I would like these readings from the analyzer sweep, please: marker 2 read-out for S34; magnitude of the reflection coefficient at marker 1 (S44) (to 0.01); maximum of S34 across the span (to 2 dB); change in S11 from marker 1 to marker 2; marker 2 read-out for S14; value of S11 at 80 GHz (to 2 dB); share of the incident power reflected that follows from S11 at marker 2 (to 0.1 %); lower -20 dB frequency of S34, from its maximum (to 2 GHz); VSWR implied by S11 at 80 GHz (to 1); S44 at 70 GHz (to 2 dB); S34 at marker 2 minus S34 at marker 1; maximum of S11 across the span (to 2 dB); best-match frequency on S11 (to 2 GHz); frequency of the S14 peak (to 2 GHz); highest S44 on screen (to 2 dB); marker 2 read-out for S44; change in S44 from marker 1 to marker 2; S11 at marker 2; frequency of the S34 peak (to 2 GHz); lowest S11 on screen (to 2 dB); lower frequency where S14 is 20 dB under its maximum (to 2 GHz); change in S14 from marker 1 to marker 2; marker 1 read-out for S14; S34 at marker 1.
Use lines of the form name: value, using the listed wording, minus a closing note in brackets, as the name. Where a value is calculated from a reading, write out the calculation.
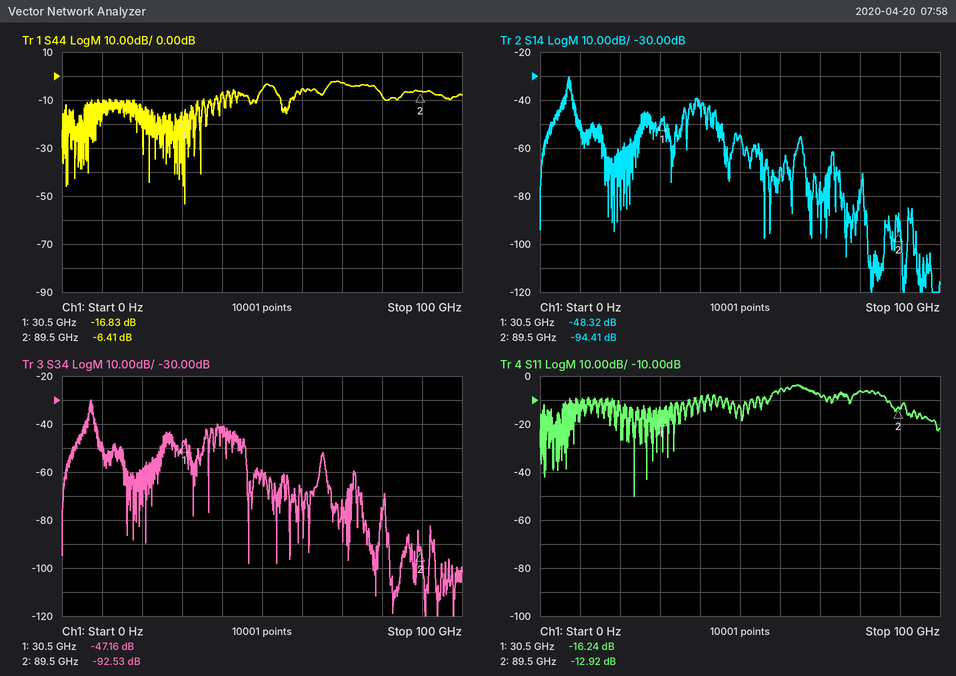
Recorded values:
marker 2 read-out for S34: -92.53 dB
magnitude of the reflection coefficient at marker 1 (S44): 10^(-16.83/20) ≈ 0.14
maximum of S34 across the span: -30 dB
change in S11 from marker 1 to marker 2: -12.92 − (-16.24) = 3.32 dB
marker 2 read-out for S14: -94.41 dB
value of S11 at 80 GHz: -6 dB
share of the incident power reflected that follows from S11 at marker 2: 10^(-12.92/10) ≈ 5.1 %
lower -20 dB frequency of S34, from its maximum: 4 GHz
VSWR implied by S11 at 80 GHz: |Γ| = 10^(-6/20) = 0.5012; VSWR = (1 + 0.5012)/(1 − 0.5012) ≈ 3
S44 at 70 GHz: -2 dB
S34 at marker 2 minus S34 at marker 1: -92.53 − (-47.16) = -45.37 dB
maximum of S11 across the span: -4 dB
best-match frequency on S11: 24 GHz
frequency of the S14 peak: 8 GHz
highest S44 on screen: -2 dB
marker 2 read-out for S44: -6.41 dB
change in S44 from marker 1 to marker 2: -6.41 − (-16.83) = 10.42 dB
S11 at marker 2: -12.92 dB
frequency of the S34 peak: 8 GHz
lowest S11 on screen: -50 dB
lower frequency where S14 is 20 dB under its maximum: 4 GHz
change in S14 from marker 1 to marker 2: -94.41 − (-48.32) = -46.09 dB
marker 1 read-out for S14: -48.32 dB
S34 at marker 1: -47.16 dB
